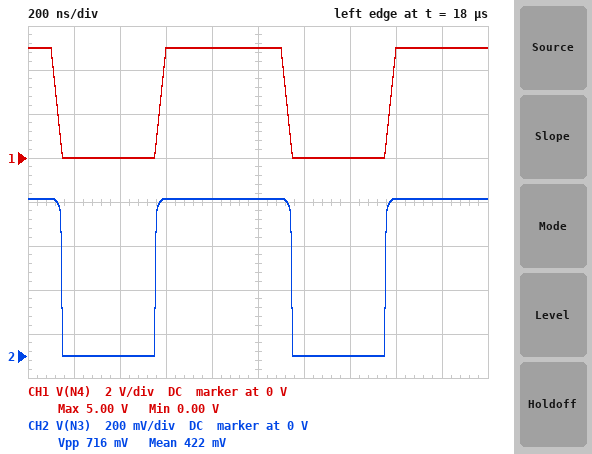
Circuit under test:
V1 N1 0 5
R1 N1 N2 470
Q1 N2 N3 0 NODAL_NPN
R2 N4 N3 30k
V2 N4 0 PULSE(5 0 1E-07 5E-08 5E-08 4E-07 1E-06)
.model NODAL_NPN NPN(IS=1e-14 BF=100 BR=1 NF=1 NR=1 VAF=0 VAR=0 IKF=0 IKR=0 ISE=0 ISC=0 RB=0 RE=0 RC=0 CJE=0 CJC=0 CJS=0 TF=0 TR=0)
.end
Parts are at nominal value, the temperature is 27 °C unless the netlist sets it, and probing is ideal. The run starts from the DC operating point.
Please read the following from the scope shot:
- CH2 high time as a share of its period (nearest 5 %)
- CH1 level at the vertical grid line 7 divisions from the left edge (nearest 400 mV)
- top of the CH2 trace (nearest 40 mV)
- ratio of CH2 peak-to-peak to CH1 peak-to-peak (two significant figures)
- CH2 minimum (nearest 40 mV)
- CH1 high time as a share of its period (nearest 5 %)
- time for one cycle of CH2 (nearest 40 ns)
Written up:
60 %
0 V
720 mV
0.14
0 V
55 %
1.00 µs
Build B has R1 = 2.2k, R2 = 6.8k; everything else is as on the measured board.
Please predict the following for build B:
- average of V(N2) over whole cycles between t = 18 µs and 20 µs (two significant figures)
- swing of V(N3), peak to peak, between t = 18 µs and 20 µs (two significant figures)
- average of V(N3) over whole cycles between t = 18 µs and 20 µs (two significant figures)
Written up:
2.1 V
690 mV
410 mV
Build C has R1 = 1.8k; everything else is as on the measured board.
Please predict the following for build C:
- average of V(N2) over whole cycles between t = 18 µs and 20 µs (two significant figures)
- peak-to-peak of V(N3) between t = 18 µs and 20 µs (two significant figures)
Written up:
2.2 V
680 mV
